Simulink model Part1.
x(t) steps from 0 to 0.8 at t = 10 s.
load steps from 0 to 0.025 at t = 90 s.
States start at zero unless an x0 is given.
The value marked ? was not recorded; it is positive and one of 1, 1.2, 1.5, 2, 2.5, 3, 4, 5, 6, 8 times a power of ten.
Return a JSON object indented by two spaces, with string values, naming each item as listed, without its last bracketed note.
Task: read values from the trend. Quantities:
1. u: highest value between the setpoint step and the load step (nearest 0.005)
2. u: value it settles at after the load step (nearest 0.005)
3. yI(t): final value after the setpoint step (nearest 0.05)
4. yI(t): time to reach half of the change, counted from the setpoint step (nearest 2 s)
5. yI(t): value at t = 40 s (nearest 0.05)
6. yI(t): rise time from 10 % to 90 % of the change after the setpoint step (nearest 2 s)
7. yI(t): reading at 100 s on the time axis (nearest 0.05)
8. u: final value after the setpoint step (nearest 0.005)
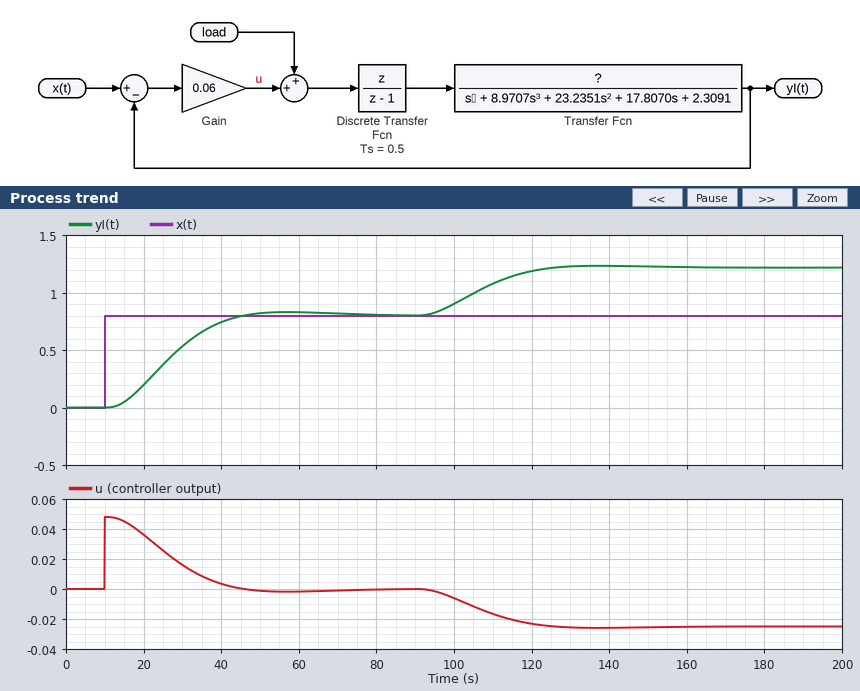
{
  "u: highest value between the setpoint step and the load step": "0.050",
  "u: value it settles at after the load step": "-0.025",
  "yI(t): final value after the setpoint step": "0.80",
  "yI(t): time to reach half of the change, counted from the setpoint step": "16 s",
  "yI(t): value at t = 40 s": "0.75",
  "yI(t): rise time from 10 % to 90 % of the change after the setpoint step": "22 s",
  "yI(t): reading at 100 s on the time axis": "0.90",
  "u: final value after the setpoint step": "0.000"
}
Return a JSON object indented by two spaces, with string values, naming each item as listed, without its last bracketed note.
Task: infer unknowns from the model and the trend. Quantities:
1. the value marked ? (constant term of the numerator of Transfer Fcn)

{
  "the value marked ?": "1.2"
}
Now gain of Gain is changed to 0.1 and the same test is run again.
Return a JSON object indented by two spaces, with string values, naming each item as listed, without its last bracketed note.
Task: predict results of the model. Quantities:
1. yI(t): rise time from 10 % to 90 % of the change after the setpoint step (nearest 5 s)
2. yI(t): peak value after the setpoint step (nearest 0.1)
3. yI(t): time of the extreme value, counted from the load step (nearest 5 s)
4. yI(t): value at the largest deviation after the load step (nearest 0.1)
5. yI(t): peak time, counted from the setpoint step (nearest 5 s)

{
  "yI(t): rise time from 10 % to 90 % of the change after the setpoint step": "15 s",
  "yI(t): peak value after the setpoint step": "0.9",
  "yI(t): time of the extreme value, counted from the load step": "30 s",
  "yI(t): value at the largest deviation after the load step": "1.1",
  "yI(t): peak time, counted from the setpoint step": "30 s"
}
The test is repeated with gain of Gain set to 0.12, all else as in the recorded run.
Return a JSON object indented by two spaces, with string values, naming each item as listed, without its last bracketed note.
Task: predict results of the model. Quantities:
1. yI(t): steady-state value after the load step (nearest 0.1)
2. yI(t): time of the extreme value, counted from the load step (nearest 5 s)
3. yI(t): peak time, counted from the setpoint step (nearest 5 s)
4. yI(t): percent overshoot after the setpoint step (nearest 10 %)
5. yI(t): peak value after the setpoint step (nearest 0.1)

{
  "yI(t): steady-state value after the load step": "1.0",
  "yI(t): time of the extreme value, counted from the load step": "25 s",
  "yI(t): peak time, counted from the setpoint step": "25 s",
  "yI(t): percent overshoot after the setpoint step": "20 %",
  "yI(t): peak value after the setpoint step": "1.0"
}
